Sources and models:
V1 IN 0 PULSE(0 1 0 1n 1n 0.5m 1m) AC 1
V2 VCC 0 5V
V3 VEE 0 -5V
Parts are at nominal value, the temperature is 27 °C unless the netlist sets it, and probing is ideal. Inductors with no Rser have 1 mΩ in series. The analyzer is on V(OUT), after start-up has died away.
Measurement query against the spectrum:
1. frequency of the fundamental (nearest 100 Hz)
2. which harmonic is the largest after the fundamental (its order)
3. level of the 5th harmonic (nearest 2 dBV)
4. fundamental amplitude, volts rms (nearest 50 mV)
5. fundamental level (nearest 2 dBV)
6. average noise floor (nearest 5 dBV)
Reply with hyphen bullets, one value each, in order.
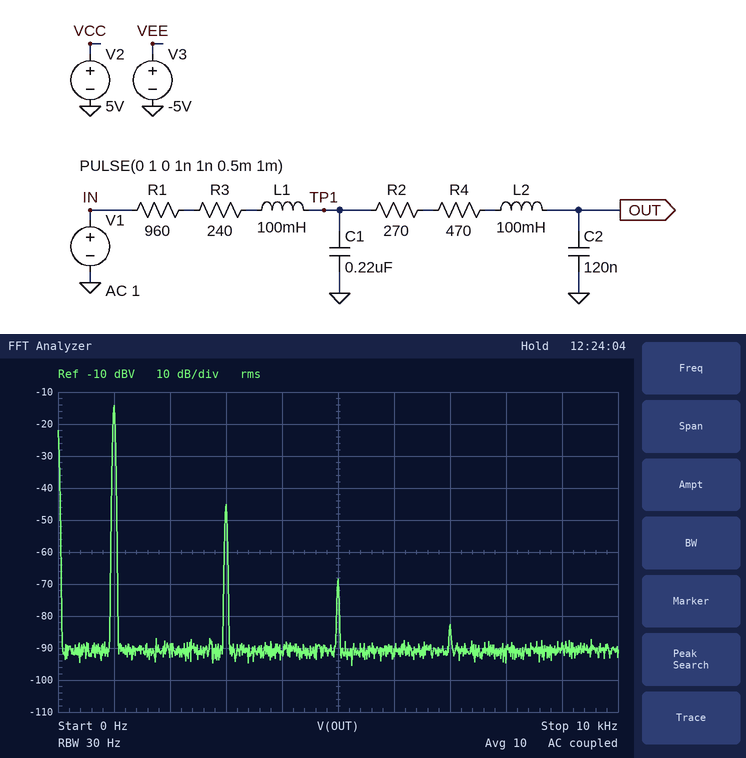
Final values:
- 1.0 kHz
- 3
- -68 dBV
- 200 mV
- -14 dBV
- -90 dBV
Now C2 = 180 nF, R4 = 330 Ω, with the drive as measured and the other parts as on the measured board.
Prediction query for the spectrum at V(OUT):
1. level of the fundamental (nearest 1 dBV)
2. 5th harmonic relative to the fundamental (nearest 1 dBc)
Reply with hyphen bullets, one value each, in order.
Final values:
- -15 dBV
- -57 dBc
